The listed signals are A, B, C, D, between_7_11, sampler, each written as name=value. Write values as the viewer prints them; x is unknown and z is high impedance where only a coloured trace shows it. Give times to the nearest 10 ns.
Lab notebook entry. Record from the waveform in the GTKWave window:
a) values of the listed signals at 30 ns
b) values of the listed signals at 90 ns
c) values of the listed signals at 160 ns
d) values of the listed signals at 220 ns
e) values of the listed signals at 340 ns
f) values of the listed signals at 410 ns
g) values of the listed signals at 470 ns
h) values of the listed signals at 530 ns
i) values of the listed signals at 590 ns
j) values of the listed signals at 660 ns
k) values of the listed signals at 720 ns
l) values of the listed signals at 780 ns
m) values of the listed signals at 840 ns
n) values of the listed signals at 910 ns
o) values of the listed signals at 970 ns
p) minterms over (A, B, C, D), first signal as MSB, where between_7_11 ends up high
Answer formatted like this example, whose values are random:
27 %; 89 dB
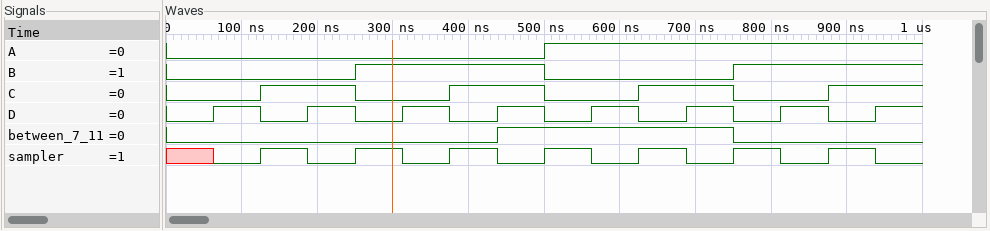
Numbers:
A=0, B=0, C=0, D=0, between_7_11=0, sampler=x; A=0, B=0, C=0, D=1, between_7_11=0, sampler=0; A=0, B=0, C=1, D=0, between_7_11=0, sampler=1; A=0, B=0, C=1, D=1, between_7_11=0, sampler=0; A=0, B=1, C=0, D=1, between_7_11=0, sampler=0; A=0, B=1, C=1, D=0, between_7_11=0, sampler=1; A=0, B=1, C=1, D=1, between_7_11=1, sampler=0; A=1, B=0, C=0, D=0, between_7_11=1, sampler=1; A=1, B=0, C=0, D=1, between_7_11=1, sampler=0; A=1, B=0, C=1, D=0, between_7_11=1, sampler=1; A=1, B=0, C=1, D=1, between_7_11=1, sampler=0; A=1, B=1, C=0, D=0, between_7_11=0, sampler=1; A=1, B=1, C=0, D=1, between_7_11=0, sampler=0; A=1, B=1, C=1, D=0, between_7_11=0, sampler=1; A=1, B=1, C=1, D=1, between_7_11=0, sampler=0; 7, 8, 9, 10, 11
